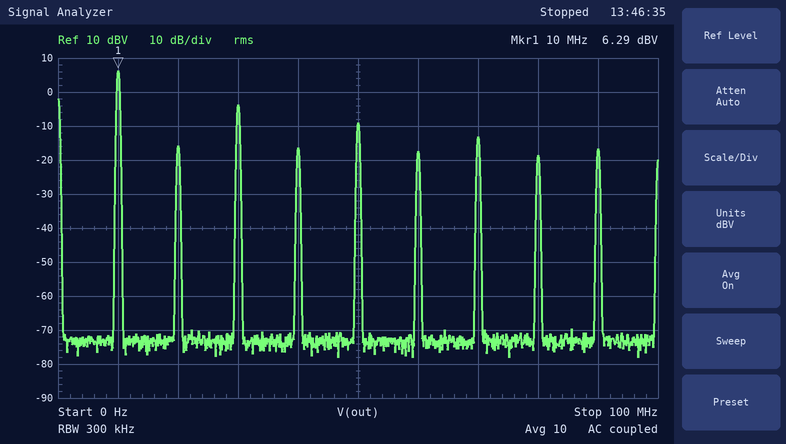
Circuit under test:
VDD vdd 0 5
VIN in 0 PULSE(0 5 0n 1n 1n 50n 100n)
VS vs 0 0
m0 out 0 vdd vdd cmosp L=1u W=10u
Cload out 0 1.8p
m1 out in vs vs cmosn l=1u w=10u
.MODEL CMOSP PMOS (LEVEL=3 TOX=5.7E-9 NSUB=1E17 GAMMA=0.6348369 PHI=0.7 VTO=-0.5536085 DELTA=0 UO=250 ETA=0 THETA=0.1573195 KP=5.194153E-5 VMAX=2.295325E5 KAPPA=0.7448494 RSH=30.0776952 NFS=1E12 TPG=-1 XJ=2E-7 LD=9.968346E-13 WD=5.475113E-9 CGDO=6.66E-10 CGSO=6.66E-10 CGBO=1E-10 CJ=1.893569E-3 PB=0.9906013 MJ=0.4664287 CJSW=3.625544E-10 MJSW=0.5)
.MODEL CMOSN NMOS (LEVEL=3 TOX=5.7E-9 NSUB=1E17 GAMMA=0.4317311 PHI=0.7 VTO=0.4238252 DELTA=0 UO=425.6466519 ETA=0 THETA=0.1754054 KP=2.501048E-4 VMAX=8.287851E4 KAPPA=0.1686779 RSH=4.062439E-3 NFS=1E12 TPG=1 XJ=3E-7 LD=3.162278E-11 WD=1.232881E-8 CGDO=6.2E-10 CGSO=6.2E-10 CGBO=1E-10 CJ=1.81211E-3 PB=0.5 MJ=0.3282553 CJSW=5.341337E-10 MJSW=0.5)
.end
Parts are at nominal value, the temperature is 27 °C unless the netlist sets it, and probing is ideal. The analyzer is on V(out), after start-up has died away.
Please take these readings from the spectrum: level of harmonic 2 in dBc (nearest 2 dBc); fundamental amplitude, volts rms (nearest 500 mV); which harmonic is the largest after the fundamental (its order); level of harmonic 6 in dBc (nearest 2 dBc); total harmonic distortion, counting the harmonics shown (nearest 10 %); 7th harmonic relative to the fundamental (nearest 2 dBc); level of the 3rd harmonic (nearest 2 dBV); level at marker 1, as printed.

-22 dBc
2.0 V
3
-24 dBc
40 %
-20 dBc
-4 dBV
6.29 dBV
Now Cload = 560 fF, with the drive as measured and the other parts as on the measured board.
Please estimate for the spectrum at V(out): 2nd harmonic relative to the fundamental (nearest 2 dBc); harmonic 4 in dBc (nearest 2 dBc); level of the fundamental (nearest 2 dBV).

-26 dBc
-26 dBc
6 dBV
